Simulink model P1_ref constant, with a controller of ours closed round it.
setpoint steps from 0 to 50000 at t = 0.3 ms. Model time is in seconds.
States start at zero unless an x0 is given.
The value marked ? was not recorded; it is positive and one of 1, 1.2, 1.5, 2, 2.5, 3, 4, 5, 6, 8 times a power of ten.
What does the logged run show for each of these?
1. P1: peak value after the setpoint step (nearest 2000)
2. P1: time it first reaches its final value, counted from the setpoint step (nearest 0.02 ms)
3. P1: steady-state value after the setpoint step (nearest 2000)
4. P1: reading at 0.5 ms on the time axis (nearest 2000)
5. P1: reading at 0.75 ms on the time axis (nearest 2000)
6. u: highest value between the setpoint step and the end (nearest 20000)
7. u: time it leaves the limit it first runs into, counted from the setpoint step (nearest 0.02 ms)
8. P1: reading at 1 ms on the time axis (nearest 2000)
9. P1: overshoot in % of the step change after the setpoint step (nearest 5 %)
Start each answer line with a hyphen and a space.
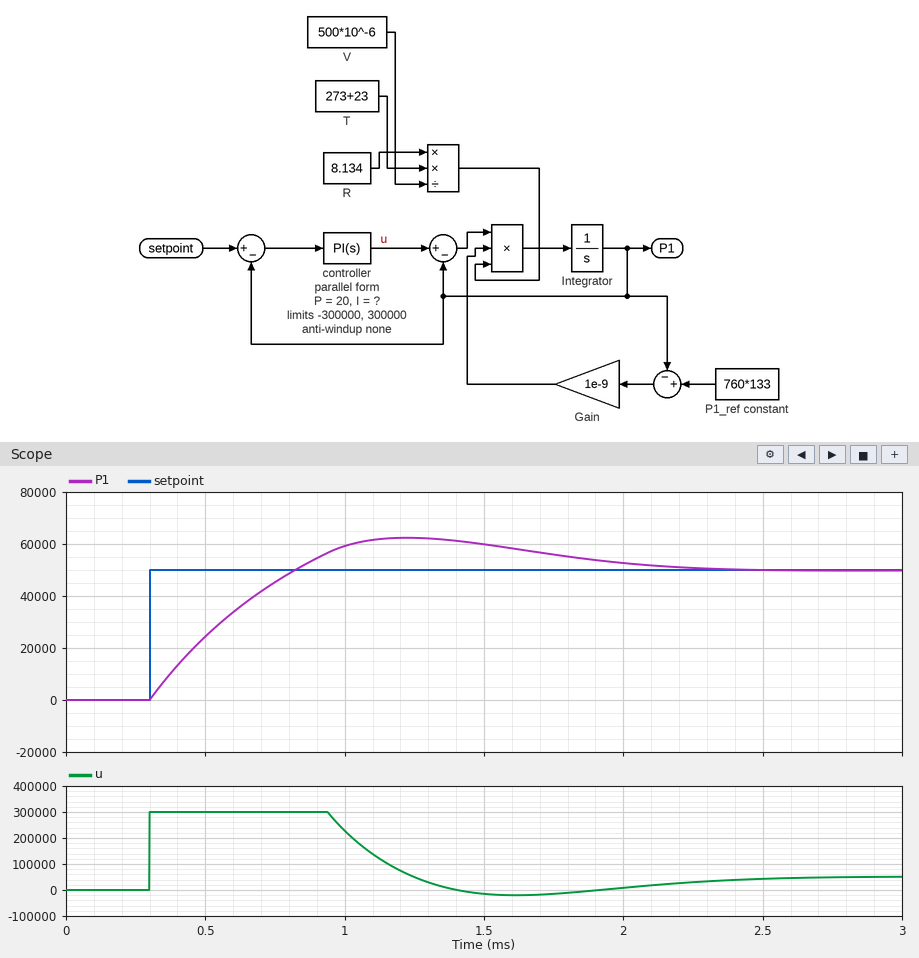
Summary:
- 62000
- 0.52 ms
- 50000
- 24000
- 46000
- 300000
- 0.64 ms
- 60000
- 25 %
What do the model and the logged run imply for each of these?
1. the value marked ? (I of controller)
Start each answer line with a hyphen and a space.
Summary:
- 40000
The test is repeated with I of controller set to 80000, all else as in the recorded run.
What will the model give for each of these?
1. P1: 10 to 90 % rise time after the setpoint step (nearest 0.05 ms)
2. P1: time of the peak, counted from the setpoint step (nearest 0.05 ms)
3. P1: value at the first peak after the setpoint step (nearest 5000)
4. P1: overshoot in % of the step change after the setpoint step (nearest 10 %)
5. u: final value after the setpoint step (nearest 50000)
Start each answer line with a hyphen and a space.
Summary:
- 0.40 ms
- 1.00 ms
- 70000
- 40 %
- 50000
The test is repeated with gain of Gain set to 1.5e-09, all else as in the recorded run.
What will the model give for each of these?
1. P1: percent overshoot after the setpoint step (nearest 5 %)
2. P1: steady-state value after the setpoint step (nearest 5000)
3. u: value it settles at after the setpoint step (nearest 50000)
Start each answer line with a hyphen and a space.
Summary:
- 15 %
- 50000
- 50000
